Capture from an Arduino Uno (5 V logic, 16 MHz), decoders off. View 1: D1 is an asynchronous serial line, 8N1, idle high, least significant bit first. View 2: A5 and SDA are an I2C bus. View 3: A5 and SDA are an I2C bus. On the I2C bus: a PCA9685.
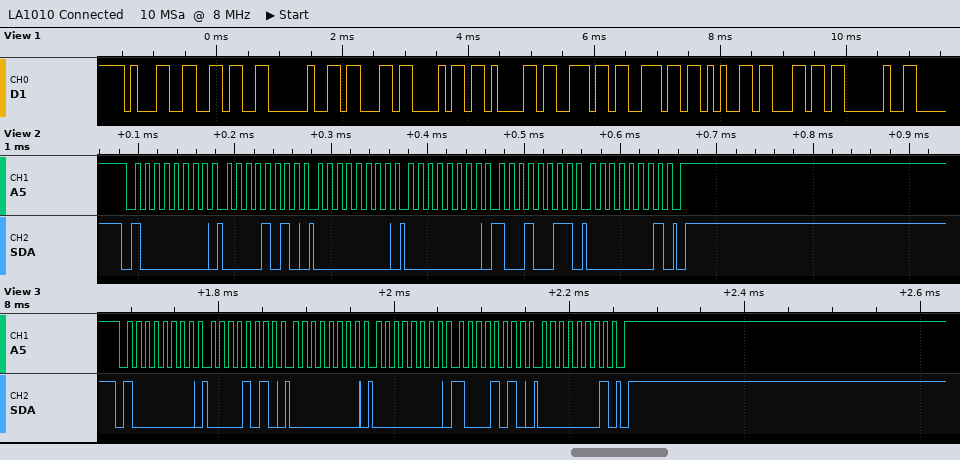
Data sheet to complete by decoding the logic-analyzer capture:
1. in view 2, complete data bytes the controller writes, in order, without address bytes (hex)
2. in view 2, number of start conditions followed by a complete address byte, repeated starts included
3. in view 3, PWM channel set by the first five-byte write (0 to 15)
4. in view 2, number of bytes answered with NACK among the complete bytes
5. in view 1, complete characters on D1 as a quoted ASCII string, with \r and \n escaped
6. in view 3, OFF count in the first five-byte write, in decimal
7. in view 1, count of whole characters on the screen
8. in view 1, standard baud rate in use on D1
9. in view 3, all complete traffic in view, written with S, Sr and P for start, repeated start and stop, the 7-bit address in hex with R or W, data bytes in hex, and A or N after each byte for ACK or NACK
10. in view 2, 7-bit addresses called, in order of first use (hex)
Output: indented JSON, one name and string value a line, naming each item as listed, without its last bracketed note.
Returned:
{
  "in view 2, complete data bytes the controller writes, in order, without address bytes": "0A 00 00 93 01",
  "in view 2, number of start conditions followed by a complete address byte, repeated starts included": "1",
  "in view 3, PWM channel set by the first five-byte write": "1",
  "in view 2, number of bytes answered with NACK among the complete bytes": "0",
  "in view 1, complete characters on D1 as a quoted ASCII string, with \\r and \\n escaped": "\"16 channel \"",
  "in view 3, OFF count in the first five-byte write, in decimal": "394",
  "in view 1, count of whole characters on the screen": "11",
  "in view 1, standard baud rate in use on D1": "9600 baud",
  "in view 3, all complete traffic in view, written with S, Sr and P for start, repeated start and stop, the 7-bit address in hex with R or W, data bytes in hex, and A or N after each byte for ACK or NACK": "S 40W A 0A A 00 A 00 A 8A A 01 A P",
  "in view 2, 7-bit addresses called, in order of first use": "0x40"
}
